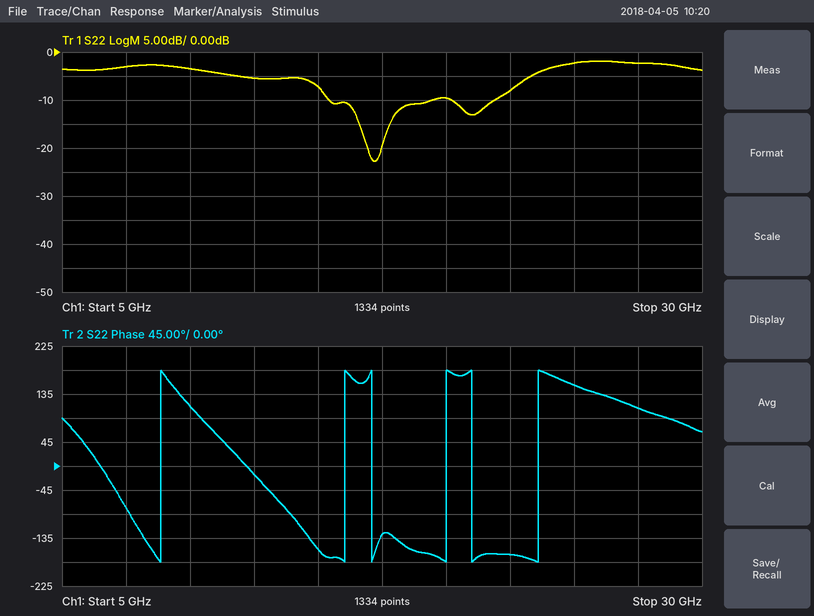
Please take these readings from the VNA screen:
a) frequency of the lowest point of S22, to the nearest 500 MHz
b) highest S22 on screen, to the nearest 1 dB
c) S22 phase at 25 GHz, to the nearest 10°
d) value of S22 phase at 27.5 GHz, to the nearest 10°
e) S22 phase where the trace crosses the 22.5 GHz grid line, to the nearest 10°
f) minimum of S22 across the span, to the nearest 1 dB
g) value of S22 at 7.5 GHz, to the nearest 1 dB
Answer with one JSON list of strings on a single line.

["17.0 GHz", "-2 dB", "150°", "110°", "-170°", "-23 dB", "-3 dB"]
